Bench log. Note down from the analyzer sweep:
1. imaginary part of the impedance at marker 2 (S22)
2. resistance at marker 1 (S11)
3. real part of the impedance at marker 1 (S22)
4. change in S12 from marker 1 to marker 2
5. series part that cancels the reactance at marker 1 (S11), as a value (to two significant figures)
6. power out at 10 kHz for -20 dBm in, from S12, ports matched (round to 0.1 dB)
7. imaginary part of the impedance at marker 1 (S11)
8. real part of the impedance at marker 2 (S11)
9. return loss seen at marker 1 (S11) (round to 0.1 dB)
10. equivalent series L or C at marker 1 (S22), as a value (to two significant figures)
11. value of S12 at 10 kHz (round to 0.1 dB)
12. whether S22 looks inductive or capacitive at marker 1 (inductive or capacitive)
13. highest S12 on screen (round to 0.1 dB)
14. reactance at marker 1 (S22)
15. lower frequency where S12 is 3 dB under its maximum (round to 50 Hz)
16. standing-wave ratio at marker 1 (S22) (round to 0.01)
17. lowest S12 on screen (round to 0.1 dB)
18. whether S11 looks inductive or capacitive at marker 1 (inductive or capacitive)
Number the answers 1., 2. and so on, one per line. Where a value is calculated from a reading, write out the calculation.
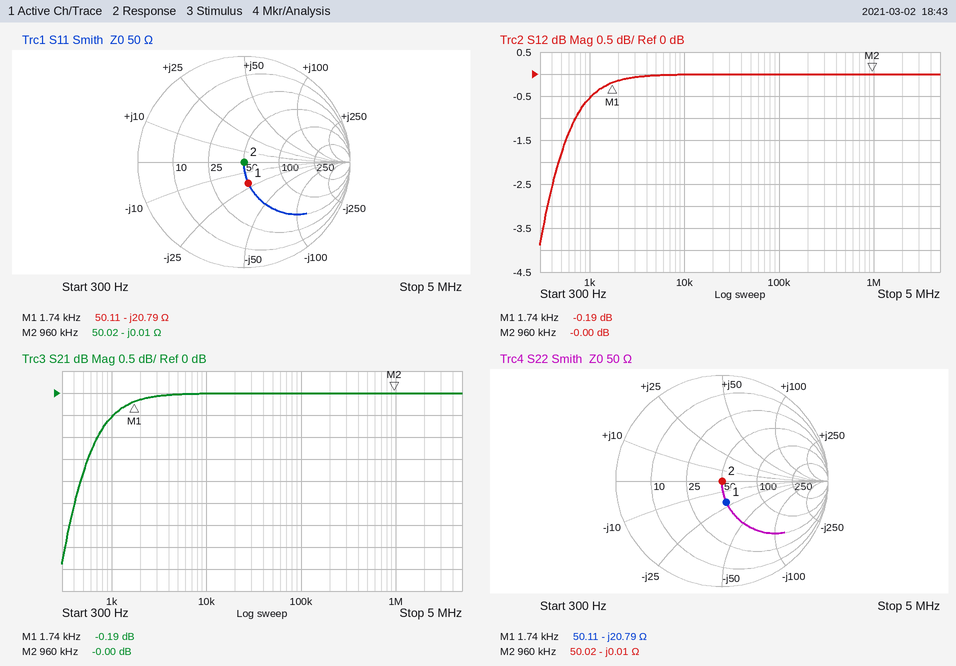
1. -0.01 Ω
2. 50.11 Ω
3. 50.11 Ω
4. -0 − (-0.19) = 0.19 dB
5. L = 20.79 Ω/(2π × 1.74 kHz) ≈ 1.9 mH
6. -20 dBm + (0.0 dB) = -20.0 dBm
7. -20.79 Ω
8. 50.02 Ω
9. 13.8 dB
10. C = 1/(2π × 1.74 kHz × 20.79 Ω) ≈ 4.4 µF
11. 0.0 dB
12. capacitive
13. 0.0 dB
14. -20.79 Ω
15. 350 Hz
16. 1.51
17. -3.9 dB
18. capacitive
